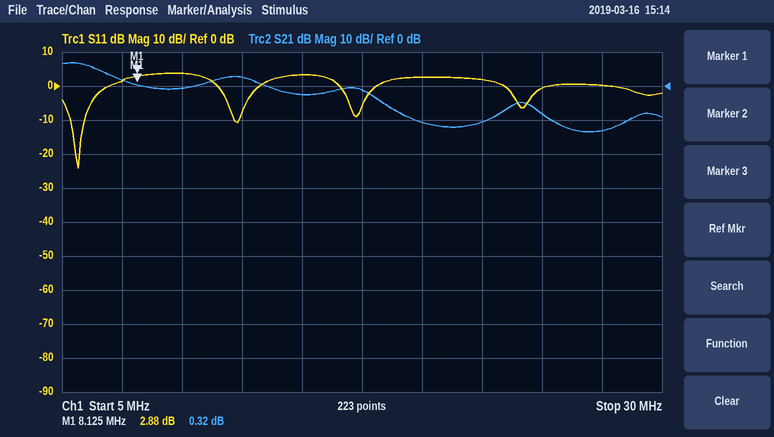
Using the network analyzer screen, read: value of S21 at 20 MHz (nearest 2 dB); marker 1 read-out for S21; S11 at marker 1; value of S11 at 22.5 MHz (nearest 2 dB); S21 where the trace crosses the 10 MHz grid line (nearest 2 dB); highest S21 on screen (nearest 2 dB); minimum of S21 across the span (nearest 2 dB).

-10 dB
0.32 dB
2.88 dB
2 dB
0 dB
6 dB
-14 dB
